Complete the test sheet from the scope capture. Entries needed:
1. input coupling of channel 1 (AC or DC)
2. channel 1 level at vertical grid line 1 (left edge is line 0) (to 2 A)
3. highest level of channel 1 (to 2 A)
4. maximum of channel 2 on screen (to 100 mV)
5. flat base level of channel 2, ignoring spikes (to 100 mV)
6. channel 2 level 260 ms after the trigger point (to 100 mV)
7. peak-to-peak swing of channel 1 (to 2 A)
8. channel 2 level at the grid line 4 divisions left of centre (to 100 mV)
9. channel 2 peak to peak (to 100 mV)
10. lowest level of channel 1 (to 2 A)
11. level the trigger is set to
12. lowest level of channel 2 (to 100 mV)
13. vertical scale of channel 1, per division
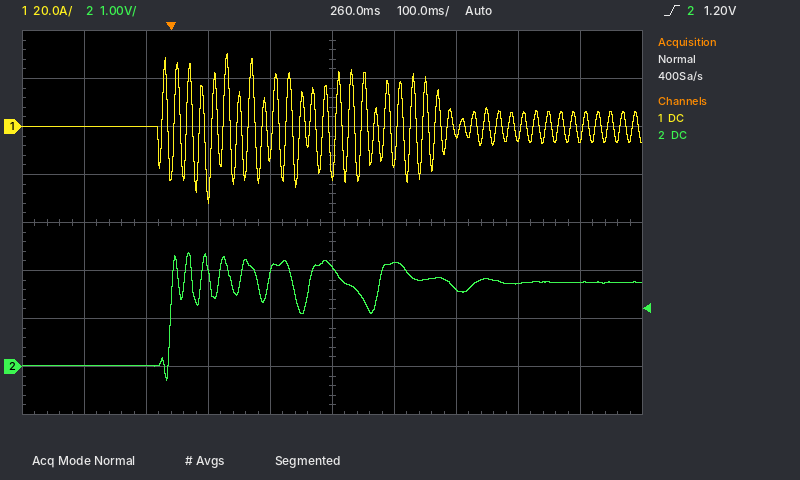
DC
0 A
30 A
2.4 V
0.0 V
2.1 V
62 A
0.0 V
2.7 V
-32 A
1.20 V
-300 mV
20 A
